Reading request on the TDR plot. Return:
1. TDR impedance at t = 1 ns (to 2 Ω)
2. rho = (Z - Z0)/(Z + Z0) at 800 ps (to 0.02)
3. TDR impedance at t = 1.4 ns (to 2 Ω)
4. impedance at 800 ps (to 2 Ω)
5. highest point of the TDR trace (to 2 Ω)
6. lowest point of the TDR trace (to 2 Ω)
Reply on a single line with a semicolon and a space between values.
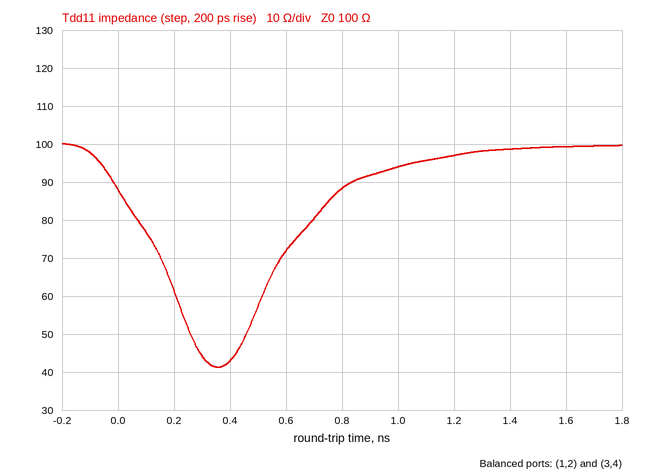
94 Ω; -0.06; 98 Ω; 88 Ω; 100 Ω; 42 Ω
